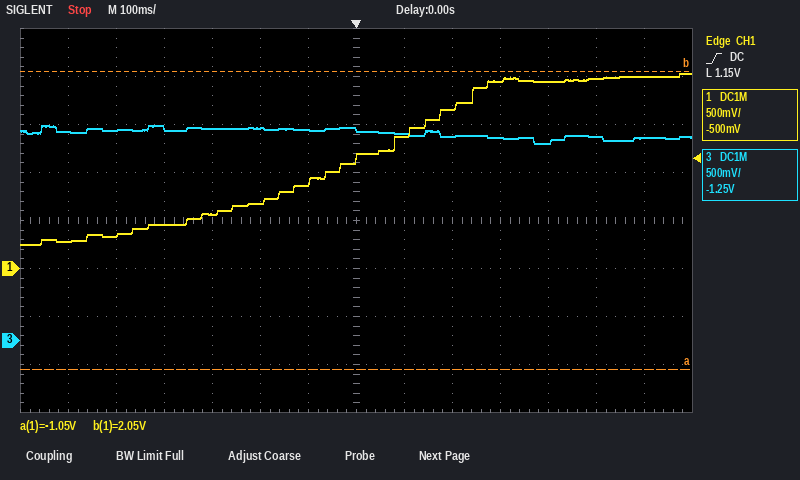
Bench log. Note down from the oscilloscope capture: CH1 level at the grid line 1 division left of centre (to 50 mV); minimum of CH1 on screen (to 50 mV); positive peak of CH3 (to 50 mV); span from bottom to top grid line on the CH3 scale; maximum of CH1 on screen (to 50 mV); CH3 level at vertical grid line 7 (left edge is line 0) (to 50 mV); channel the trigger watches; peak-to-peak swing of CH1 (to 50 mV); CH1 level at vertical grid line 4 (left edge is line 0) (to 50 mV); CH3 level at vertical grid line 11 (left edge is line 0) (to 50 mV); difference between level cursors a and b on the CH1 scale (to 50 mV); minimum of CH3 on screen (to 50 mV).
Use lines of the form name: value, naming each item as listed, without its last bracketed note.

CH1 level at the grid line 1 division left of centre: 900 mV
minimum of CH1 on screen: 250 mV
positive peak of CH3: 2.25 V
span from bottom to top grid line on the CH3 scale: 4 V
maximum of CH1 on screen: 2.05 V
CH3 level at vertical grid line 7 (left edge is line 0): 2.20 V
channel the trigger watches: CH1
peak-to-peak swing of CH1: 1.80 V
CH1 level at vertical grid line 4 (left edge is line 0): 550 mV
CH3 level at vertical grid line 11 (left edge is line 0): 2.05 V
difference between level cursors a and b on the CH1 scale: 3.10 V
minimum of CH3 on screen: 2.05 V
